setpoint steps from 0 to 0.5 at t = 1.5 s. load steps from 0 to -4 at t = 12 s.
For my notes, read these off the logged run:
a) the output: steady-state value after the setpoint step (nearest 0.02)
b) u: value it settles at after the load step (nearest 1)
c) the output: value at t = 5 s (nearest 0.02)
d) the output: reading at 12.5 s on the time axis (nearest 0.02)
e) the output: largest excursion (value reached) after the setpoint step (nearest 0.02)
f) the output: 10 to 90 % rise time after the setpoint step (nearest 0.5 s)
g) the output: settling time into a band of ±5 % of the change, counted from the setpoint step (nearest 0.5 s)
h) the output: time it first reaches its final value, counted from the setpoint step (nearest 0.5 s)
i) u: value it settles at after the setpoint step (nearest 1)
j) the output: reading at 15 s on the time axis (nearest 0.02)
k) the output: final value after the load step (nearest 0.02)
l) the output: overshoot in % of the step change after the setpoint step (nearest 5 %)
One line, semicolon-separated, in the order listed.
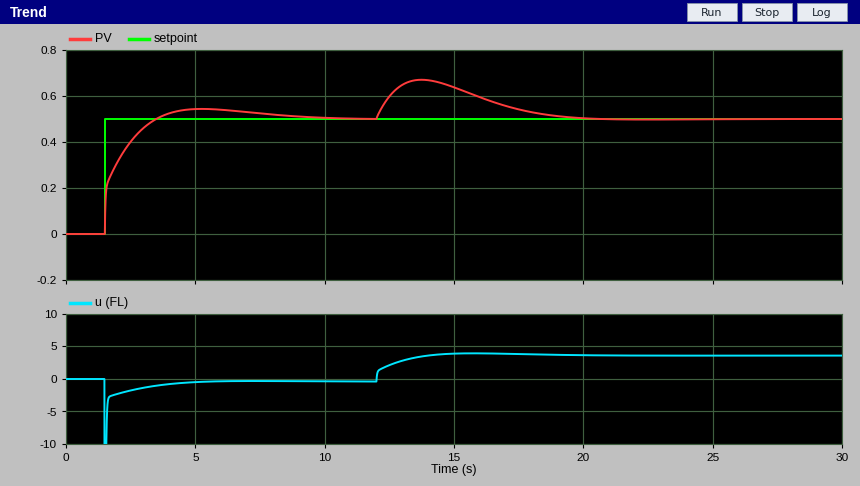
0.50; 4; 0.54; 0.60; 0.54; 1.5 s; 6.0 s; 2.0 s; 0; 0.64; 0.50; 10 %
